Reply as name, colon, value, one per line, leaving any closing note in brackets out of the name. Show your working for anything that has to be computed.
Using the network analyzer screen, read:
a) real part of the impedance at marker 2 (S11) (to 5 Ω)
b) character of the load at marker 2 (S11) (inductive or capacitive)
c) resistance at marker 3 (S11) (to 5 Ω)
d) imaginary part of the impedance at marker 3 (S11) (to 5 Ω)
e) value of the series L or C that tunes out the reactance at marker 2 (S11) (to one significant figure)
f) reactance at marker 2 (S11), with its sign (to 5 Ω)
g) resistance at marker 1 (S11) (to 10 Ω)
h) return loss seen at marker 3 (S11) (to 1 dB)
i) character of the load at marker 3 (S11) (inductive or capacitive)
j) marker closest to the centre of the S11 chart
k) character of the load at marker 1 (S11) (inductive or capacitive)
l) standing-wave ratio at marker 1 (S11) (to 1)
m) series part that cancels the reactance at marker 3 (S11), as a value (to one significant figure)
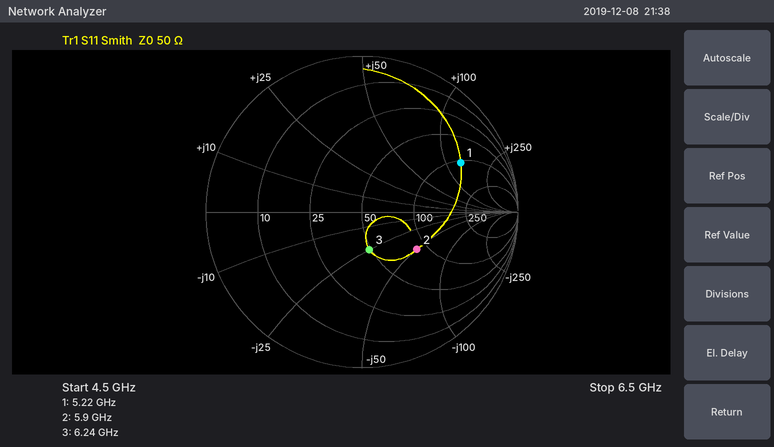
real part of the impedance at marker 2 (S11): 85 Ω
character of the load at marker 2 (S11): capacitive
resistance at marker 3 (S11): 50 Ω
imaginary part of the impedance at marker 3 (S11): -25 Ω
value of the series L or C that tunes out the reactance at marker 2 (S11): L = 50 Ω/(2π × 5.9 GHz) ≈ 1 nH
reactance at marker 2 (S11), with its sign: -50 Ω
resistance at marker 1 (S11): 110 Ω
return loss seen at marker 3 (S11): 12 dB
character of the load at marker 3 (S11): capacitive
marker closest to the centre of the S11 chart: marker 3
character of the load at marker 1 (S11): inductive
standing-wave ratio at marker 1 (S11): 6
series part that cancels the reactance at marker 3 (S11), as a value: L = 25 Ω/(2π × 6.24 GHz) ≈ 638 pH, so 600 pH to one significant figure
